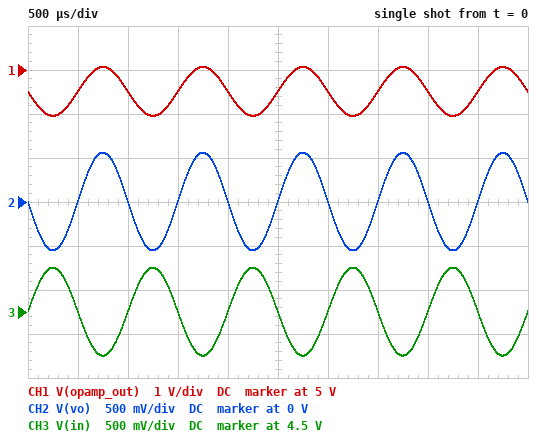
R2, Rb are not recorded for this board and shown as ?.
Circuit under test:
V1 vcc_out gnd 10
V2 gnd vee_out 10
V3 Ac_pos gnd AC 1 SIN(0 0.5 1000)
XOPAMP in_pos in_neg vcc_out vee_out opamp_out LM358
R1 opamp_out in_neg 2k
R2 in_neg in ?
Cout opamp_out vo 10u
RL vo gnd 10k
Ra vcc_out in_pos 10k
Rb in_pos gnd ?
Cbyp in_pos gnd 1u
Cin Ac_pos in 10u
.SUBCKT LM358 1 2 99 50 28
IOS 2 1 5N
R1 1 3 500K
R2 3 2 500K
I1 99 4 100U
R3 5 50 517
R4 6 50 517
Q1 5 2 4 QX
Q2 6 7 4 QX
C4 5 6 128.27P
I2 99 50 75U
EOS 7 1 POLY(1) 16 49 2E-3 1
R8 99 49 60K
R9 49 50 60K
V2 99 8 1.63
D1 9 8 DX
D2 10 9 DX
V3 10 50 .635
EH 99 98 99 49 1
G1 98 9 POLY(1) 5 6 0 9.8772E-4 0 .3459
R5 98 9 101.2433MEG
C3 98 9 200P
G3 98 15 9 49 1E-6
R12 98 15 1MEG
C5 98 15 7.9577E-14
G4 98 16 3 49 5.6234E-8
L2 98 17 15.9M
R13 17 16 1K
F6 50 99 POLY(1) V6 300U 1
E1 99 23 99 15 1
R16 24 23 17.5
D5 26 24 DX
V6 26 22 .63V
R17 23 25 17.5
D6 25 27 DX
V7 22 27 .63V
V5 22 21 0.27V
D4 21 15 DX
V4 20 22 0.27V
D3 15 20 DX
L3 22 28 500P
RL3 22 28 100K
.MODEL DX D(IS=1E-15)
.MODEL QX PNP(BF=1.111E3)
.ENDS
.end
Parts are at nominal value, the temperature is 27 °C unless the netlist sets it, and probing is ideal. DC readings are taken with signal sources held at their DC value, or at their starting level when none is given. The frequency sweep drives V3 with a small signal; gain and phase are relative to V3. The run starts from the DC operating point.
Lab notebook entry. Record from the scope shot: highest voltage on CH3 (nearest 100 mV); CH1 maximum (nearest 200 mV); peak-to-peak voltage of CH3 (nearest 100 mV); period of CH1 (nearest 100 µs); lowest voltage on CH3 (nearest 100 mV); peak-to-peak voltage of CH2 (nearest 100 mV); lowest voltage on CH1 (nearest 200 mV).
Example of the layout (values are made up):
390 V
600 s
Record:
5.0 V
5.0 V
1.0 V
1.0 ms
4.0 V
1.1 V
4.0 V
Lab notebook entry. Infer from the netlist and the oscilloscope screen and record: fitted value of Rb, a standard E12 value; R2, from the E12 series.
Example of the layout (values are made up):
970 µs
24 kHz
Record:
8.2 kΩ
1.8 kΩ
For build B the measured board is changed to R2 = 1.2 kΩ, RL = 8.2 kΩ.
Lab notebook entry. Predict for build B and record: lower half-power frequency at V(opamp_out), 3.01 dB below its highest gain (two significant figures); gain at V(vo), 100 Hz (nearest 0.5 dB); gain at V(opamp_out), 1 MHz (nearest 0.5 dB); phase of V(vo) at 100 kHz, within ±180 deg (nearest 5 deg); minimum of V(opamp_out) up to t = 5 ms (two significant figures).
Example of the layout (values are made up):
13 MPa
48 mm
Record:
13 Hz
4.5 dB
-7.0 dB
155 deg
3.7 V
